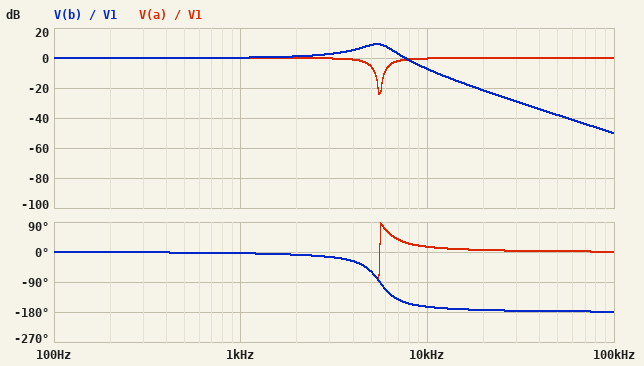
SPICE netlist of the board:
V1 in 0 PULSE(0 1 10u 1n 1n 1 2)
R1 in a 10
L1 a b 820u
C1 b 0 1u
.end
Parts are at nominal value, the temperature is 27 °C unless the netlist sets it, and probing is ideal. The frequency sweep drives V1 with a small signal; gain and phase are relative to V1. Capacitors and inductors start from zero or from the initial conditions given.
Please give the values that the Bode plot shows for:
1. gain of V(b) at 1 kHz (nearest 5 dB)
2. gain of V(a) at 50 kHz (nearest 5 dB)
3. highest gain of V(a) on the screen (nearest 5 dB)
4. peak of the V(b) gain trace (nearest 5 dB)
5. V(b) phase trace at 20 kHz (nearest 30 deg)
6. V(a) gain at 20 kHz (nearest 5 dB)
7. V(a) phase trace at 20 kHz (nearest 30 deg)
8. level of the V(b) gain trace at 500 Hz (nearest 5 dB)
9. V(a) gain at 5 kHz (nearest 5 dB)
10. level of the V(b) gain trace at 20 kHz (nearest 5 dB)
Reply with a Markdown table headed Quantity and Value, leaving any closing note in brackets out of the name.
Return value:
| Quantity | Value |
|---|---|
| gain of V(b) at 1 kHz | 0 dB |
| gain of V(a) at 50 kHz | 0 dB |
| highest gain of V(a) on the screen | 0 dB |
| peak of the V(b) gain trace | 10 dB |
| V(b) phase trace at 20 kHz | -180 deg |
| V(a) gain at 20 kHz | 0 dB |
| V(a) phase trace at 20 kHz | 0 deg |
| level of the V(b) gain trace at 500 Hz | 0 dB |
| V(a) gain at 5 kHz | -5 dB |
| level of the V(b) gain trace at 20 kHz | -20 dB |
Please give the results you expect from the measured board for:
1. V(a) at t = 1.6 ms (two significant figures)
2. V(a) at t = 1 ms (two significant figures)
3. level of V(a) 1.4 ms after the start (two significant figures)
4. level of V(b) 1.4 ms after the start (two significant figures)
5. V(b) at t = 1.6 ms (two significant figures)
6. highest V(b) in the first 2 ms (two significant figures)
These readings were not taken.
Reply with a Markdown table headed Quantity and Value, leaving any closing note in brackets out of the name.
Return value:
| Quantity | Value |
|---|---|
| V(a) at t = 1.6 ms | 1.0 V |
| V(a) at t = 1 ms | 1.0 V |
| level of V(a) 1.4 ms after the start | 1.0 V |
| level of V(b) 1.4 ms after the start | 1.0 V |
| V(b) at t = 1.6 ms | 1.0 V |
| highest V(b) in the first 2 ms | 1.6 V |
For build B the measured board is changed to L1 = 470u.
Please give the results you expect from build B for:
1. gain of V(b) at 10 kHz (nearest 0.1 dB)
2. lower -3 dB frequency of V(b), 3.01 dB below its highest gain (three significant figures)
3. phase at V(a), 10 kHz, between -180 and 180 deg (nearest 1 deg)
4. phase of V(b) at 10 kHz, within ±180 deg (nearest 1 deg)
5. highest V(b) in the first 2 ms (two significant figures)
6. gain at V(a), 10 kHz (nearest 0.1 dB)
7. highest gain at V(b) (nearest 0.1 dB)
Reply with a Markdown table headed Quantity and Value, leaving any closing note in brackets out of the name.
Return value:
| Quantity | Value |
|---|---|
| gain of V(b) at 10 kHz | -0.5 dB |
| lower -3 dB frequency of V(b), 3.01 dB below its highest gain | 4.90 kHz |
| phase at V(a), 10 kHz, between -180 and 180 deg | 36 deg |
| phase of V(b) at 10 kHz, within ±180 deg | -144 deg |
| highest V(b) in the first 2 ms | 1.5 V |
| gain at V(a), 10 kHz | -1.9 dB |
| highest gain at V(b) | 7.0 dB |
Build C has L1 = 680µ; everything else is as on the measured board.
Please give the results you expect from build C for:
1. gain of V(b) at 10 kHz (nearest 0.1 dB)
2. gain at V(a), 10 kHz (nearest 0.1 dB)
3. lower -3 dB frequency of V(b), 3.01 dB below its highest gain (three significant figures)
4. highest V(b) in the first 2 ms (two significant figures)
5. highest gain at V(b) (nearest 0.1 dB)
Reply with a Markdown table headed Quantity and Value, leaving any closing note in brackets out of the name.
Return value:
| Quantity | Value |
|---|---|
| gain of V(b) at 10 kHz | -5.1 dB |
| gain at V(a), 10 kHz | -0.6 dB |
| lower -3 dB frequency of V(b), 3.01 dB below its highest gain | 4.53 kHz |
| highest V(b) in the first 2 ms | 1.5 V |
| highest gain at V(b) | 8.5 dB |
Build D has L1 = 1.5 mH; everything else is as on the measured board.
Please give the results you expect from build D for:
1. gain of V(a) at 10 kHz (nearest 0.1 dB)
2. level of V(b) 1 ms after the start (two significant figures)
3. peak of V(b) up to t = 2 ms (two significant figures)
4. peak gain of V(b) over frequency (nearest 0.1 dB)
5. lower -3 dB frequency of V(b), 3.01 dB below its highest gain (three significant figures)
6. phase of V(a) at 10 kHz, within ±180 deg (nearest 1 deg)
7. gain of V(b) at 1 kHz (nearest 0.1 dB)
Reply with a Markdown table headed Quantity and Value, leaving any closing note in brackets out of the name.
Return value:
| Quantity | Value |
|---|---|
| gain of V(a) at 10 kHz | -0.1 dB |
| level of V(b) 1 ms after the start | 960 mV |
| peak of V(b) up to t = 2 ms | 1.7 V |
| peak gain of V(b) over frequency | 11.8 dB |
| lower -3 dB frequency of V(b), 3.01 dB below its highest gain | 3.46 kHz |
| phase of V(a) at 10 kHz, within ±180 deg | 7 deg |
| gain of V(b) at 1 kHz | 0.5 dB |
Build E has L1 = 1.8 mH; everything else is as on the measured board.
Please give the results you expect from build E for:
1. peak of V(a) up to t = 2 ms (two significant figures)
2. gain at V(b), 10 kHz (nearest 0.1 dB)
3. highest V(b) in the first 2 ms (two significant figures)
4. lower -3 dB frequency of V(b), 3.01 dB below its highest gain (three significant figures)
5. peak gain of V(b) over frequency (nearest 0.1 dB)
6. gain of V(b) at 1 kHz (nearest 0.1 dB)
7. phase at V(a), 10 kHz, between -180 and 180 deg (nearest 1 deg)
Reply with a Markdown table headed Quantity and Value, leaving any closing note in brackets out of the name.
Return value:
| Quantity | Value |
|---|---|
| peak of V(a) up to t = 2 ms | 1.1 V |
| gain at V(b), 10 kHz | -15.8 dB |
| highest V(b) in the first 2 ms | 1.7 V |
| lower -3 dB frequency of V(b), 3.01 dB below its highest gain | 3.22 kHz |
| peak gain of V(b) over frequency | 12.6 dB |
| gain of V(b) at 1 kHz | 0.6 dB |
| phase at V(a), 10 kHz, between -180 and 180 deg | 6 deg |
